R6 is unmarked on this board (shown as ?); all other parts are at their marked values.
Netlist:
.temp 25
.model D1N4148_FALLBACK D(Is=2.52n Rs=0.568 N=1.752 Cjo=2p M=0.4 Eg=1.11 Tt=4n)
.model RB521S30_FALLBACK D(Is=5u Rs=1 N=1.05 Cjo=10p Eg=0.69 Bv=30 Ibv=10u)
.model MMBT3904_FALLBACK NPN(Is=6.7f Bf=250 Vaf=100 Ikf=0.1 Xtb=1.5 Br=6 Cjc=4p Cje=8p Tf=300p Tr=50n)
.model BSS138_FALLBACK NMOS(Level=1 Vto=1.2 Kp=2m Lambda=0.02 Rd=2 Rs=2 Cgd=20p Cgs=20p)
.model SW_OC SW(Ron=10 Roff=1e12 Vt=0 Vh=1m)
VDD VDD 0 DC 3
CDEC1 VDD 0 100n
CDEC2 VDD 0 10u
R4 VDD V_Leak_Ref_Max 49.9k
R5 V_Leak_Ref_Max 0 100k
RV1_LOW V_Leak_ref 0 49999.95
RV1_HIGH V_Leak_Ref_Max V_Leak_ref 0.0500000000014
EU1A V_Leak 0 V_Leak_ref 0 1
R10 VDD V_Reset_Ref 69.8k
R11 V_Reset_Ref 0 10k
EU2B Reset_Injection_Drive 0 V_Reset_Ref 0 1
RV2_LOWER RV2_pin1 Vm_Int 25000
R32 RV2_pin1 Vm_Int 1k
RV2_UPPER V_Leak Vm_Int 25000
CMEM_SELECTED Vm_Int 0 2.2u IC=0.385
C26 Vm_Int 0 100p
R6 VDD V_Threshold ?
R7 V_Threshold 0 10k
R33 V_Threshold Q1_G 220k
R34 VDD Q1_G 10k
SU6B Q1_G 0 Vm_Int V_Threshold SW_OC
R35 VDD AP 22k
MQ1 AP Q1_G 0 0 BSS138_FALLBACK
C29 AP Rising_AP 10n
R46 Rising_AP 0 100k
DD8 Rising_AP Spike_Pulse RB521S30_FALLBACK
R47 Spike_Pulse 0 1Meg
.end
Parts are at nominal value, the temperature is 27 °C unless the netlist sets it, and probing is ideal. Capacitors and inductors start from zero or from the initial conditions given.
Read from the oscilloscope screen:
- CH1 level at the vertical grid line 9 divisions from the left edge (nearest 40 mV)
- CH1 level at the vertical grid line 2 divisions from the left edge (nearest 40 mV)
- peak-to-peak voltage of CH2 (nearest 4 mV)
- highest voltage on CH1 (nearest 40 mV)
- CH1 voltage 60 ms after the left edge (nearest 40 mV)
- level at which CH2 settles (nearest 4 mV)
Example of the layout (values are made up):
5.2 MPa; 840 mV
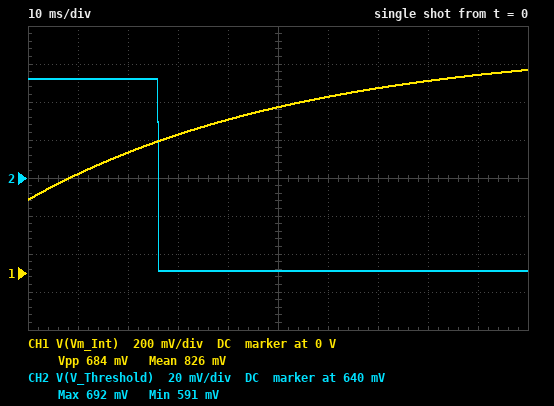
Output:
1.04 V; 640 mV; 100 mV; 1.08 V; 920 mV; 592 mV
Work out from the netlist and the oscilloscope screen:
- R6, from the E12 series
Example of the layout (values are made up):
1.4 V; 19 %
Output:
39 kΩ
